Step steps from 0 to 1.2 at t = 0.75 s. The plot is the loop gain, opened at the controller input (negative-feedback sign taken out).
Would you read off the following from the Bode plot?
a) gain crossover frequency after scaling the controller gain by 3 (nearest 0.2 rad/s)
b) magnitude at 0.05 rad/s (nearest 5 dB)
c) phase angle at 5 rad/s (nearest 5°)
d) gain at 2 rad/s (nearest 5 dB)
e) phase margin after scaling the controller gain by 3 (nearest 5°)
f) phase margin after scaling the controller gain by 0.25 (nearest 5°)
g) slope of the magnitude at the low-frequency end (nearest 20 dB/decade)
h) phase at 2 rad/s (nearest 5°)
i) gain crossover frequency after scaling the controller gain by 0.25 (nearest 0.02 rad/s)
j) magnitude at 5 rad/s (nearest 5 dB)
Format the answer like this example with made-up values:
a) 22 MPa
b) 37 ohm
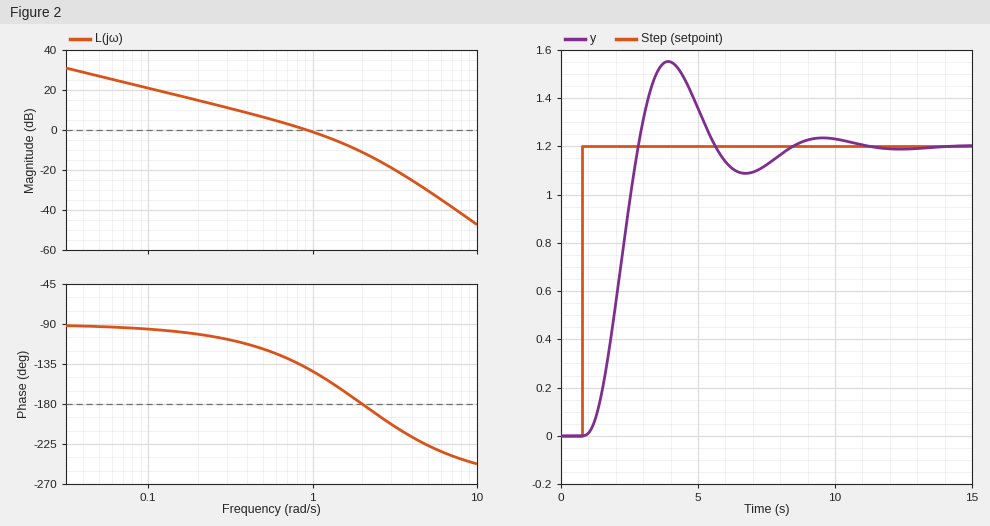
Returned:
a) 1.8 rad/s
b) 25 dB
c) -225°
d) -10 dB
e) 5°
f) 75°
g) -20 dB/decade
h) -180°
i) 0.28 rad/s
j) -30 dB
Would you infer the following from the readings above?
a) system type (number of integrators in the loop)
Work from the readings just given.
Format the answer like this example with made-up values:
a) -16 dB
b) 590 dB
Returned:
a) 1
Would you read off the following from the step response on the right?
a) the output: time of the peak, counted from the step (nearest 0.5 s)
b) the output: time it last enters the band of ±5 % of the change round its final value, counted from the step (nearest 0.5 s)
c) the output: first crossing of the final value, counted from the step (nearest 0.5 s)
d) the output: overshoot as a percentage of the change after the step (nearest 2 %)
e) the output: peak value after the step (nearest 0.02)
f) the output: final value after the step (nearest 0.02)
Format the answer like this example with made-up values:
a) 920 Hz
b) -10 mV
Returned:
a) 3.0 s
b) 7.0 s
c) 2.0 s
d) 30 %
e) 1.56
f) 1.20
